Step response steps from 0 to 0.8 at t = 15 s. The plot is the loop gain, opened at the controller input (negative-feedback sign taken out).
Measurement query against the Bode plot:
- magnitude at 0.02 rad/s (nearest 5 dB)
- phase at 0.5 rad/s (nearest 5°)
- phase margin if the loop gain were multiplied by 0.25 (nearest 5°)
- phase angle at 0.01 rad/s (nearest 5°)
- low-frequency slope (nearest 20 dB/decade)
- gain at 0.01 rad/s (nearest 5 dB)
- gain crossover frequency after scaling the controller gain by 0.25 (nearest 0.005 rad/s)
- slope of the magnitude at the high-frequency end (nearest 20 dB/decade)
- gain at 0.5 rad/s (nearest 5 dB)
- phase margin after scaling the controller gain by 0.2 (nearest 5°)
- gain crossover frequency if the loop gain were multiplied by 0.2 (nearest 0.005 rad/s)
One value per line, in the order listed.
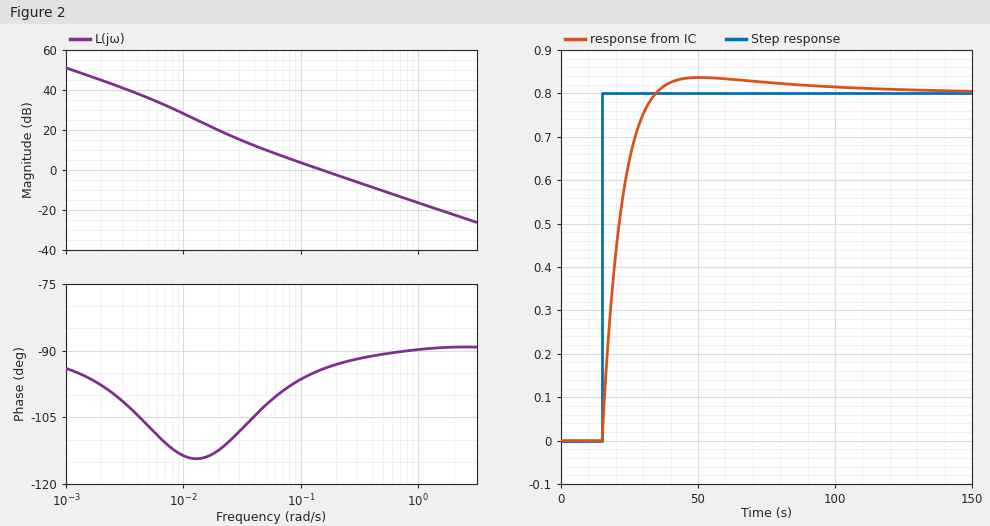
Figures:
20 dB
-90°
75°
-115°
-20 dB/decade
30 dB
0.040 rad/s
-20 dB/decade
-10 dB
75°
0.035 rad/s
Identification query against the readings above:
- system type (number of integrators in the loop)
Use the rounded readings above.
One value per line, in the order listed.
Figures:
1
